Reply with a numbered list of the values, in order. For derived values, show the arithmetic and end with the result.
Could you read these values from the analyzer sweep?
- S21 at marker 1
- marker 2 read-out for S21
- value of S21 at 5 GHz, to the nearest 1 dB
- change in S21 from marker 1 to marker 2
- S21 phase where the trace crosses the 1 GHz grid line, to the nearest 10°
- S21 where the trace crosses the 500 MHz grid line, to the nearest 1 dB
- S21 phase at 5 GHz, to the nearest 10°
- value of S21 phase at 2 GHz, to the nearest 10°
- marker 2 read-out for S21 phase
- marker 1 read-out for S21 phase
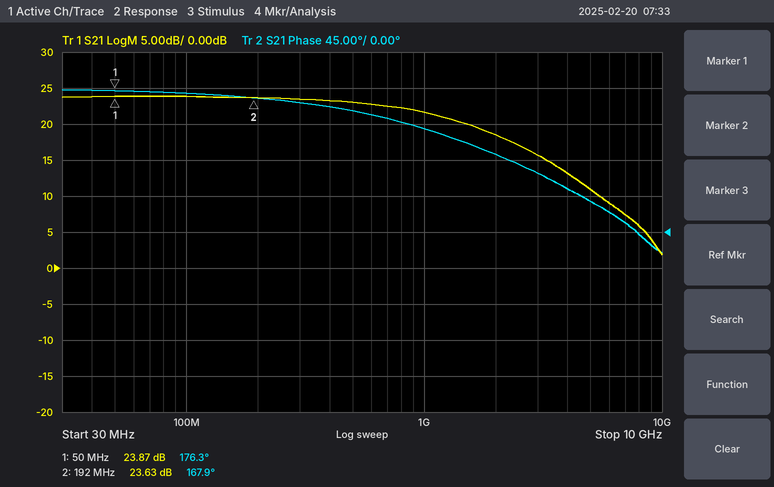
1. 23.87 dB
2. 23.63 dB
3. 11 dB
4. 23.63 − (23.87) = -0.24 dB
5. 130°
6. 23 dB
7. 40°
8. 100°
9. 167.9°
10. 176.3°
